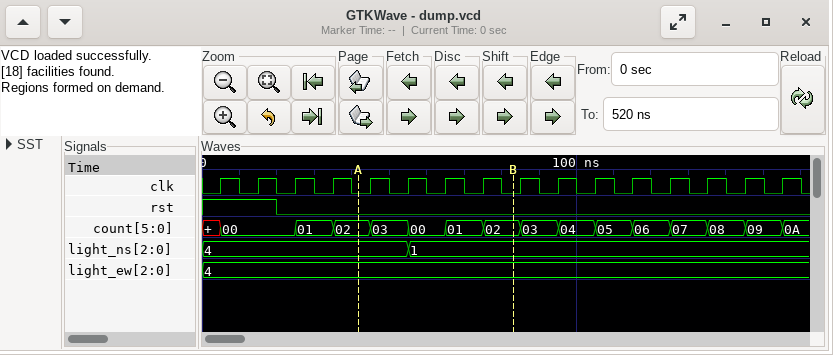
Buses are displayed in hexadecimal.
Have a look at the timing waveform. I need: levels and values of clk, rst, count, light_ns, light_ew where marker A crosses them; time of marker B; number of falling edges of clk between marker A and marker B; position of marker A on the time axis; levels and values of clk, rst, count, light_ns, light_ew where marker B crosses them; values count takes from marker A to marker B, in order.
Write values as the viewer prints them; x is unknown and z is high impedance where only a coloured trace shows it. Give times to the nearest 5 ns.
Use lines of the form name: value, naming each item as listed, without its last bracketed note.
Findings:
levels and values of clk, rst, count, light_ns, light_ew where marker A crosses them: clk=0, rst=0, count=02, light_ns=4, light_ew=4
time of marker B: 85 ns
number of falling edges of clk between marker A and marker B: 4
position of marker A on the time axis: 40 ns
levels and values of clk, rst, count, light_ns, light_ew where marker B crosses them: clk=0, rst=0, count=02, light_ns=1, light_ew=4
values count takes from marker A to marker B, in order: 02, 03, 00, 01, 02
